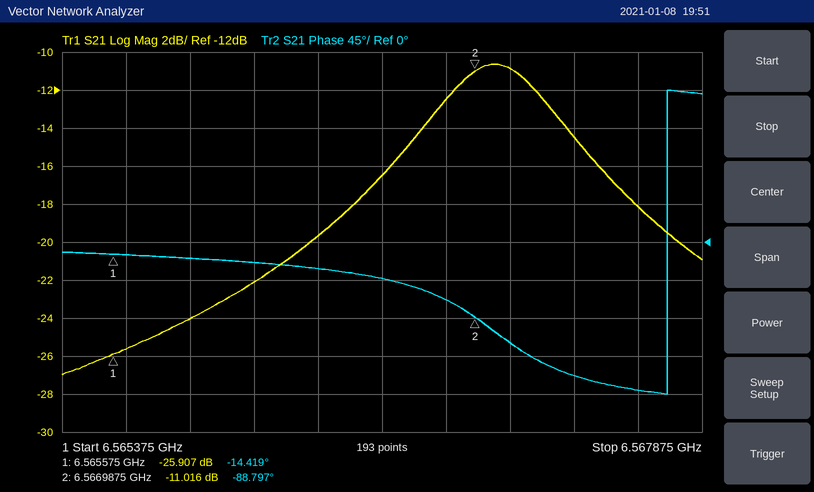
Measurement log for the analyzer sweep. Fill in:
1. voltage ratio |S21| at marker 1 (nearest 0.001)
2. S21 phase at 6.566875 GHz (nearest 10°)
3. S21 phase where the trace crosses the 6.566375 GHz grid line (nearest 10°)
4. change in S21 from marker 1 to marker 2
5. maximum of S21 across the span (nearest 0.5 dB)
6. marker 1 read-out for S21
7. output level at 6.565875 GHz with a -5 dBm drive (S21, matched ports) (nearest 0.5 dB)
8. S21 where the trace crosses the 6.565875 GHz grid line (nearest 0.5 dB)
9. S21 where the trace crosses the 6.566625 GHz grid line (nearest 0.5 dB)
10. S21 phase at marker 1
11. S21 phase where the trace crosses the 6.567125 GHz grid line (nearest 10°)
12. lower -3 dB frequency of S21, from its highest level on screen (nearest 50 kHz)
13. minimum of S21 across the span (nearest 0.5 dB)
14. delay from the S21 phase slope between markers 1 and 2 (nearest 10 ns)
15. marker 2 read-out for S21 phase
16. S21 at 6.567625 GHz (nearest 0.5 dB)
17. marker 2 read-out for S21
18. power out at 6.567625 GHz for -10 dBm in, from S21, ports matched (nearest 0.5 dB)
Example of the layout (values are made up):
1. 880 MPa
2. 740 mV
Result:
1. 0.051
2. -70°
3. -30°
4. 14.891 dB
5. -10.5 dB
6. -25.907 dB
7. -29.0 dBm
8. -24.0 dB
9. -16.5 dB
10. -14.419°
11. -120°
12. 6.56680 GHz
13. -27.0 dB
14. 150 ns
15. -88.797°
16. -18.0 dB
17. -11.016 dB
18. -28.0 dBm
